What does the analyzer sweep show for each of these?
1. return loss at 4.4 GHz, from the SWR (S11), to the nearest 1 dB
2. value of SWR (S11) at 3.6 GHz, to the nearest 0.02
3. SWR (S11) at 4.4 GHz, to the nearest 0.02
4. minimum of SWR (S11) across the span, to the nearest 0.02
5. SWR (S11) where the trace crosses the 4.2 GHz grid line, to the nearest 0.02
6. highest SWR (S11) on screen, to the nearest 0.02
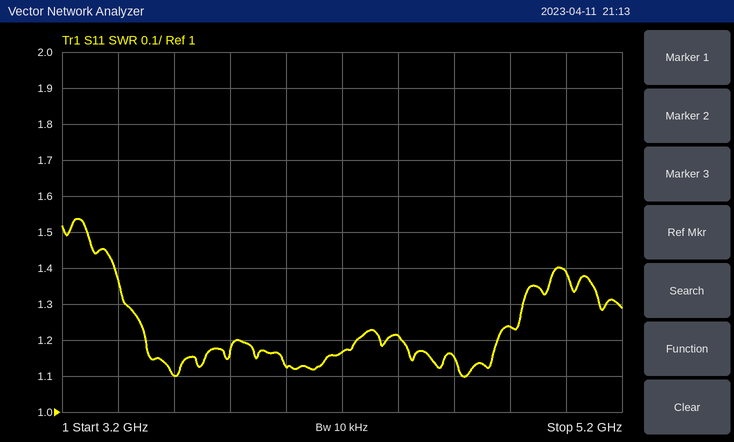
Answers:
20 dB
1.10
1.22
1.10
1.16
1.54
